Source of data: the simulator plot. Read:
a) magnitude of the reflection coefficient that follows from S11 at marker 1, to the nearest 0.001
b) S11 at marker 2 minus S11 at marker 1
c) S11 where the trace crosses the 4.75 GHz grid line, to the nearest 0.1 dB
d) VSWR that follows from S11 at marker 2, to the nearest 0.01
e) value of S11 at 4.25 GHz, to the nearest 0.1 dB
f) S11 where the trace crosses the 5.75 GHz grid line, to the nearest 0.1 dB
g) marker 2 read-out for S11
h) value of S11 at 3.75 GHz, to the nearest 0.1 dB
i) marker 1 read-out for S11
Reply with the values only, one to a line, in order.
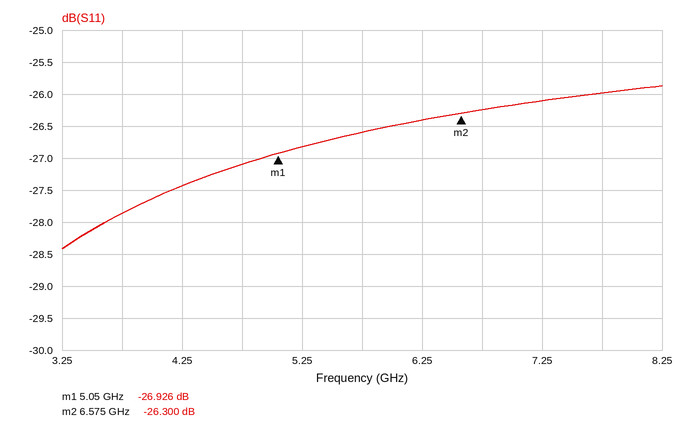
0.045
0.626 dB
-27.1 dB
1.10
-27.4 dB
-26.6 dB
-26.300 dB
-27.9 dB
-26.926 dB
